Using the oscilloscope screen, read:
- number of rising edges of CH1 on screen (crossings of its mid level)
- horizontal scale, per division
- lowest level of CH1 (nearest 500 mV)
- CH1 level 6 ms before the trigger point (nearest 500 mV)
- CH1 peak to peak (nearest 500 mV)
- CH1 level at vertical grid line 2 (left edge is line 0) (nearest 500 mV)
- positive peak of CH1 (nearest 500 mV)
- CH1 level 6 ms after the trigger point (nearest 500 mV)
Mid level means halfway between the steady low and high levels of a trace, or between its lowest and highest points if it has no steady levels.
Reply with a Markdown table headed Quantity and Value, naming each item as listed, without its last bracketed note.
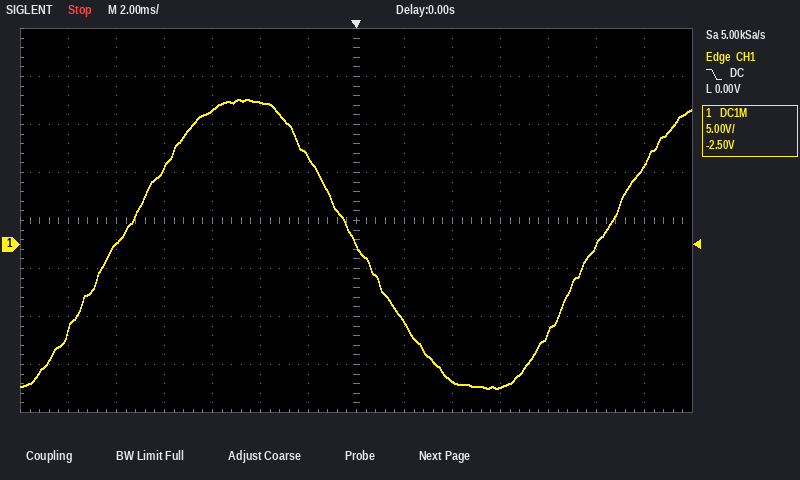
| Quantity | Value |
|---|---|
| number of rising edges of CH1 on screen | 2 |
| horizontal scale, per division | 2 ms |
| lowest level of CH1 | -15.0 V |
| CH1 level 6 ms before the trigger point | 14.0 V |
| CH1 peak to peak | 30.0 V |
| CH1 level at vertical grid line 2 (left edge is line 0) | 0.0 V |
| positive peak of CH1 | 15.0 V |
| CH1 level 6 ms after the trigger point | -15.0 V |
